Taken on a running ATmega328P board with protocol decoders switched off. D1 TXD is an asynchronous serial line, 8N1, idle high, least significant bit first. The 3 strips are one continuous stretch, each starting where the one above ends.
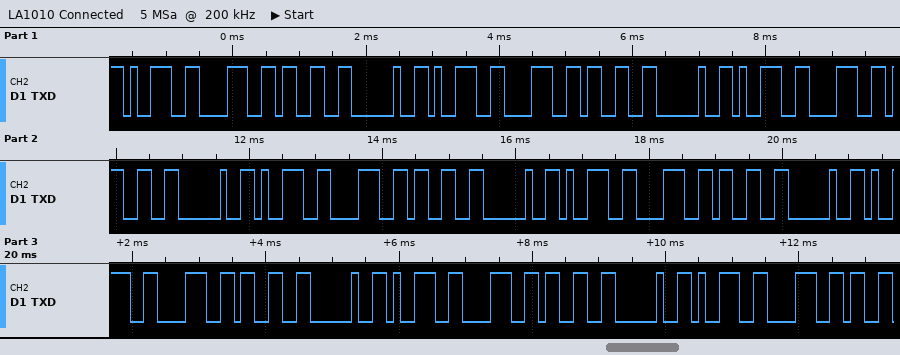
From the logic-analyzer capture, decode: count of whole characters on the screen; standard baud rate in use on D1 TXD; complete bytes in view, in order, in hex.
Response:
30
9600 baud
0x39 0x38 0x33 0x20 0x39 0x38 0x33 0x20 0x39 0x38 0x33 0x20 0x39 0x38 0x33 0x20 0x39 0x38 0x33 0x20 0x39 0x38 0x33 0x20 0x39 0x38 0x33 0x20 0x39 0x38
